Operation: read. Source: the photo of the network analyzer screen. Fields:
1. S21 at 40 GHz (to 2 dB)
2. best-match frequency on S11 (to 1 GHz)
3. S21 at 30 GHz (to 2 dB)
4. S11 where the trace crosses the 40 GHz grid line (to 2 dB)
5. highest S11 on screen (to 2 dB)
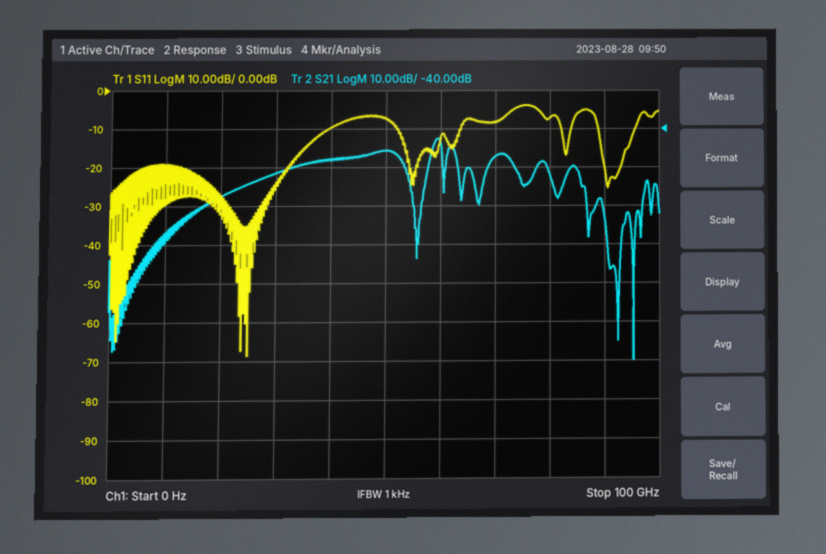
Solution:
-48 dB
25 GHz
-52 dB
-10 dB
-4 dB
